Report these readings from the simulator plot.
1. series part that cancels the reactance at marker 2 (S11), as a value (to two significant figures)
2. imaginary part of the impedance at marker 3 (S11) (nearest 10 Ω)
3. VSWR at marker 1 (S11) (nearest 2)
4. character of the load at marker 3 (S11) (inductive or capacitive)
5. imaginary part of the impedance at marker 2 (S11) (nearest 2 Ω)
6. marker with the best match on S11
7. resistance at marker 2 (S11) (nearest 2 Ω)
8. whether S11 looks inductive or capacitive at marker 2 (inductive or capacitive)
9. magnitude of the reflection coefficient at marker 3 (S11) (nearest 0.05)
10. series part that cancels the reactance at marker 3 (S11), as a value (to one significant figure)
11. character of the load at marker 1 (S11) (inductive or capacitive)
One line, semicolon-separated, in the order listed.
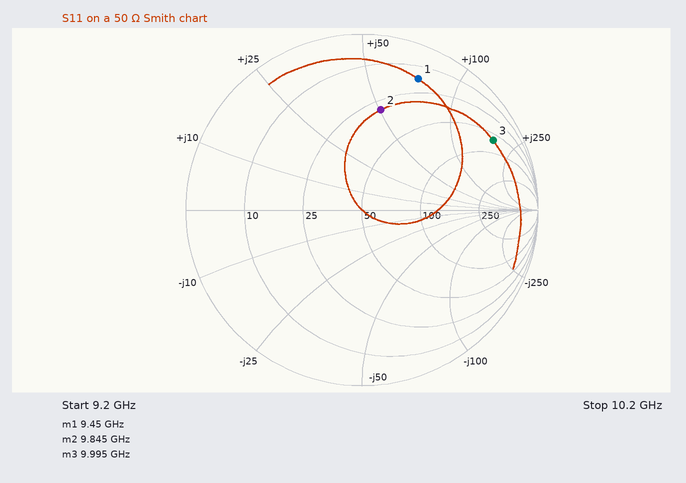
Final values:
320 fF; +180 Ω; 10; inductive; +50 Ω; marker 2; 30 Ω; inductive; 0.85; 90 fF; inductive
